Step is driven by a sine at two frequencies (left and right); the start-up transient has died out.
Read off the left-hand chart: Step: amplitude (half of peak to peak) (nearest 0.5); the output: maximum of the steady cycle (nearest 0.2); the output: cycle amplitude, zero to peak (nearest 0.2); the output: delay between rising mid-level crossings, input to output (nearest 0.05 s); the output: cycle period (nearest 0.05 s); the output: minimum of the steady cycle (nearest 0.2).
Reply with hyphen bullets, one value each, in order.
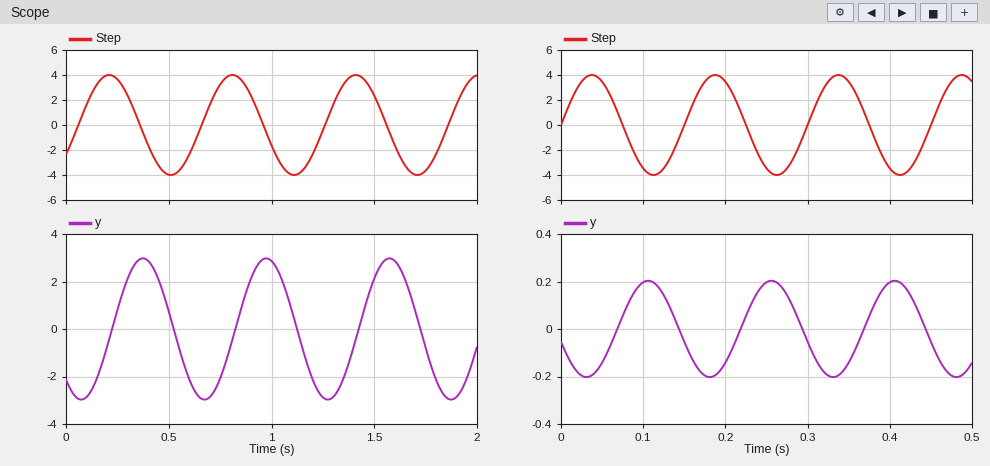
- 4.0
- 3.0
- 3.0
- 0.15 s
- 0.60 s
- -3.0
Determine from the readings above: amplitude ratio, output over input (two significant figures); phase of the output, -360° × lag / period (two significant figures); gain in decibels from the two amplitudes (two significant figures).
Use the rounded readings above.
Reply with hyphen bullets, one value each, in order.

- 0.75
- -90°
- -2.5 dB
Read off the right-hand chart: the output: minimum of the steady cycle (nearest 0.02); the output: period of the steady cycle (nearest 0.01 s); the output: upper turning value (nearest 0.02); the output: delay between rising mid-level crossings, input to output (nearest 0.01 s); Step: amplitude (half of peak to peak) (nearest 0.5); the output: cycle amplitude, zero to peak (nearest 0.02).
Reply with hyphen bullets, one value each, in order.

- -0.20
- 0.15 s
- 0.20
- 0.07 s
- 4.0
- 0.20
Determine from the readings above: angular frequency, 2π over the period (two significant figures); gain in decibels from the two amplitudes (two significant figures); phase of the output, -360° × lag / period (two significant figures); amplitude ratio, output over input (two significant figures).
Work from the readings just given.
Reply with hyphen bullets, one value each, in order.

- 42 rad/s
- -26 dB
- -170°
- 0.050
